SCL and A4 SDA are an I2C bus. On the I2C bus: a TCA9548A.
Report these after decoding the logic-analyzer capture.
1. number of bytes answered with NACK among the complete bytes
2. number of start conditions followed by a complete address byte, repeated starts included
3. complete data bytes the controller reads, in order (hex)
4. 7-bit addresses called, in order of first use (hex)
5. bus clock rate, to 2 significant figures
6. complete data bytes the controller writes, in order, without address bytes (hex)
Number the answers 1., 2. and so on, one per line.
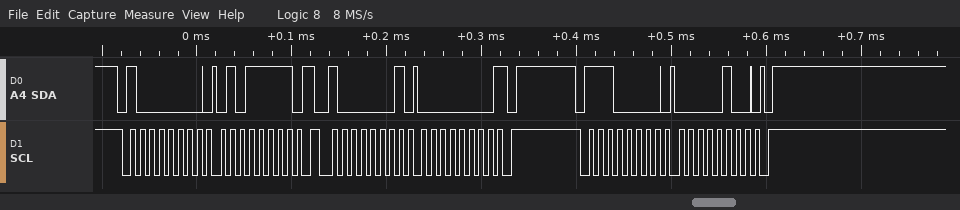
1. 1
2. 3
3. 00
4. 0x40 0x70
5. 100 kHz
6. 5F 04
